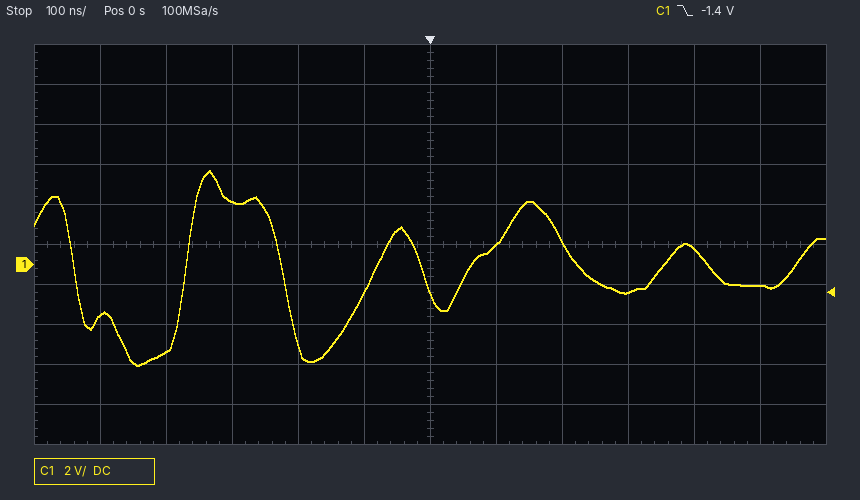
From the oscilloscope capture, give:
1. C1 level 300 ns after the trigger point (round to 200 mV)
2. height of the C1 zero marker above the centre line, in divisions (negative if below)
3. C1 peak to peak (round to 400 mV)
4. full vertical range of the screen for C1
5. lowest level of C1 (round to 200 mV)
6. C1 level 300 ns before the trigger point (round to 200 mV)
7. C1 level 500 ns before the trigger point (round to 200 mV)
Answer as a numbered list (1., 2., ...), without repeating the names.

1. -1.4 V
2. -0.5 div
3. 9.6 V
4. 20 V
5. -5.0 V
6. 3.2 V
7. -2.6 V
